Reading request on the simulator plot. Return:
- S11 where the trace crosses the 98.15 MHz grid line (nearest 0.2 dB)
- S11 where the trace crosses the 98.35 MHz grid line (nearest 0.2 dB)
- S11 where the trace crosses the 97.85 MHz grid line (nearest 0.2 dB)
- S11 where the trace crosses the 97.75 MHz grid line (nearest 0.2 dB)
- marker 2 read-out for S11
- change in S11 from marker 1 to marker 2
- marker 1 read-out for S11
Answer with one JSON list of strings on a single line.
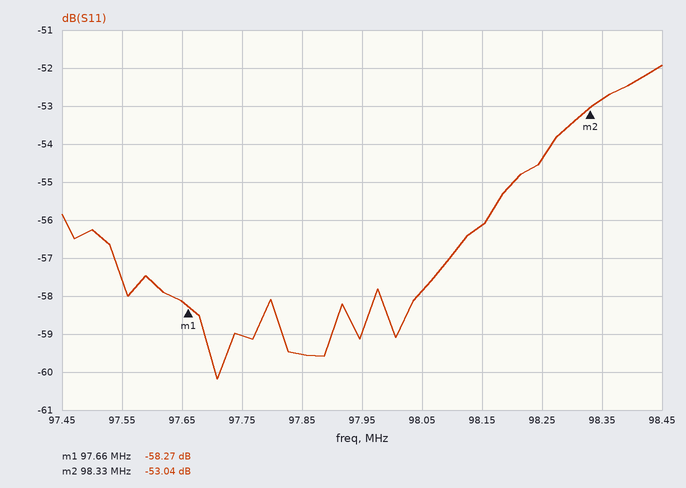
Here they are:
["-56.2 dB", "-52.8 dB", "-59.6 dB", "-59.0 dB", "-53.04 dB", "5.23 dB", "-58.27 dB"]
